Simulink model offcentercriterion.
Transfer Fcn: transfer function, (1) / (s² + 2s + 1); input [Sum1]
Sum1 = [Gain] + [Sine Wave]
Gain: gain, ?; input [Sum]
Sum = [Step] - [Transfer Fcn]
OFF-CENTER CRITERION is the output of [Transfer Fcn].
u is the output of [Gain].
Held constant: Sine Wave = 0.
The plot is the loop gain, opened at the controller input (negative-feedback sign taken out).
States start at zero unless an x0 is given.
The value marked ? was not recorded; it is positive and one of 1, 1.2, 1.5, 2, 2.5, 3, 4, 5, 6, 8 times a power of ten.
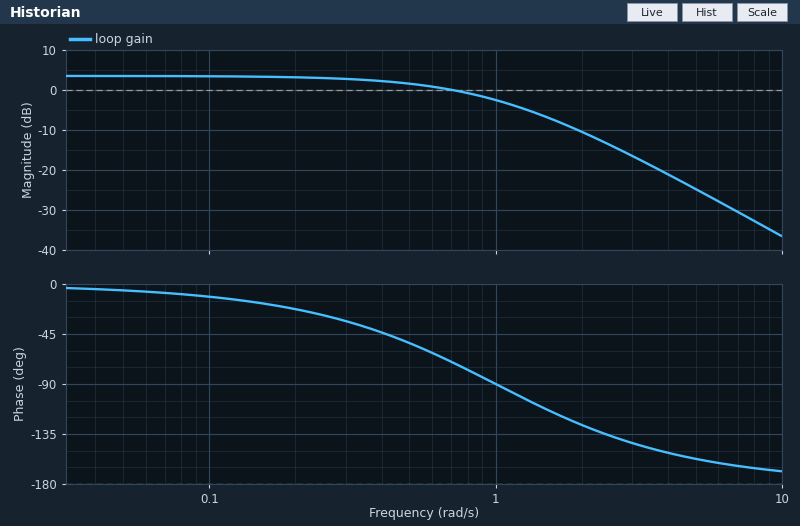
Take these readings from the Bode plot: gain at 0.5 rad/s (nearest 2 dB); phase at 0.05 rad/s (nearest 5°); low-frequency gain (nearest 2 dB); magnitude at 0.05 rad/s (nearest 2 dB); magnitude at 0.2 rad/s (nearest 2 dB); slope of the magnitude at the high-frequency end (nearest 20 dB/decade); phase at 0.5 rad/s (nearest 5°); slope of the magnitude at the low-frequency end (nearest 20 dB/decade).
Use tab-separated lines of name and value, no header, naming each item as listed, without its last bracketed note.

gain at 0.5 rad/s	2 dB
phase at 0.05 rad/s	-5°
low-frequency gain	4 dB
magnitude at 0.05 rad/s	4 dB
magnitude at 0.2 rad/s	4 dB
slope of the magnitude at the high-frequency end	-40 dB/decade
phase at 0.5 rad/s	-55°
slope of the magnitude at the low-frequency end	0 dB/decade
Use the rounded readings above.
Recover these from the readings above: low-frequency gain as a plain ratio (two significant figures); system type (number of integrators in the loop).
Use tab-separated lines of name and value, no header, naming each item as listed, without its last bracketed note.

low-frequency gain as a plain ratio	1.6
system type	0
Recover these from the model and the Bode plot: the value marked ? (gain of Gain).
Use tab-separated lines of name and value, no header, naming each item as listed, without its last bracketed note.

the value marked ?	1.5
